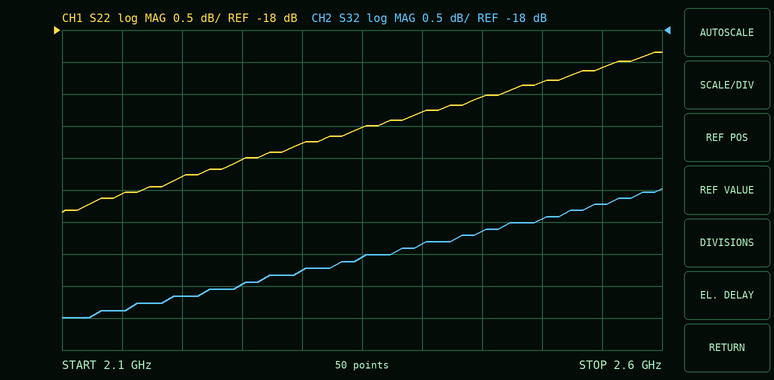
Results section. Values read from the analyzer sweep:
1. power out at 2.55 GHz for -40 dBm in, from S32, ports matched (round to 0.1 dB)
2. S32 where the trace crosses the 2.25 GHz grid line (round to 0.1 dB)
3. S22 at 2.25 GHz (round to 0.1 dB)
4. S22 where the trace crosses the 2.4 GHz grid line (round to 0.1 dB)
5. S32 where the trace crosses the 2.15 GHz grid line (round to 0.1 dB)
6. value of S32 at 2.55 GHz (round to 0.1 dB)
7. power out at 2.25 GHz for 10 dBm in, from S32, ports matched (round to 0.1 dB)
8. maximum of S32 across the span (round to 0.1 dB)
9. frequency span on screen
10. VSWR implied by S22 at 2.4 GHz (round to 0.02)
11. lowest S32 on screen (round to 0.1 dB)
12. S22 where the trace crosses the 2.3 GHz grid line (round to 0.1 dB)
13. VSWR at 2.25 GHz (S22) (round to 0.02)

-60.7 dBm
-22.0 dB
-20.0 dB
-19.3 dB
-22.4 dB
-20.7 dB
-12.0 dBm
-20.5 dB
500 MHz
1.24
-22.5 dB
-19.8 dB
1.22
